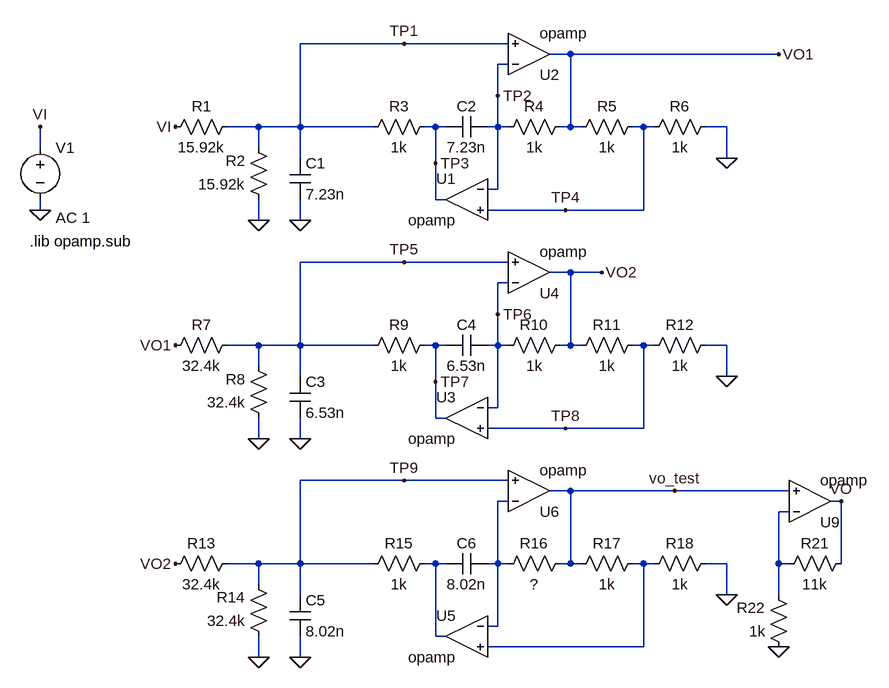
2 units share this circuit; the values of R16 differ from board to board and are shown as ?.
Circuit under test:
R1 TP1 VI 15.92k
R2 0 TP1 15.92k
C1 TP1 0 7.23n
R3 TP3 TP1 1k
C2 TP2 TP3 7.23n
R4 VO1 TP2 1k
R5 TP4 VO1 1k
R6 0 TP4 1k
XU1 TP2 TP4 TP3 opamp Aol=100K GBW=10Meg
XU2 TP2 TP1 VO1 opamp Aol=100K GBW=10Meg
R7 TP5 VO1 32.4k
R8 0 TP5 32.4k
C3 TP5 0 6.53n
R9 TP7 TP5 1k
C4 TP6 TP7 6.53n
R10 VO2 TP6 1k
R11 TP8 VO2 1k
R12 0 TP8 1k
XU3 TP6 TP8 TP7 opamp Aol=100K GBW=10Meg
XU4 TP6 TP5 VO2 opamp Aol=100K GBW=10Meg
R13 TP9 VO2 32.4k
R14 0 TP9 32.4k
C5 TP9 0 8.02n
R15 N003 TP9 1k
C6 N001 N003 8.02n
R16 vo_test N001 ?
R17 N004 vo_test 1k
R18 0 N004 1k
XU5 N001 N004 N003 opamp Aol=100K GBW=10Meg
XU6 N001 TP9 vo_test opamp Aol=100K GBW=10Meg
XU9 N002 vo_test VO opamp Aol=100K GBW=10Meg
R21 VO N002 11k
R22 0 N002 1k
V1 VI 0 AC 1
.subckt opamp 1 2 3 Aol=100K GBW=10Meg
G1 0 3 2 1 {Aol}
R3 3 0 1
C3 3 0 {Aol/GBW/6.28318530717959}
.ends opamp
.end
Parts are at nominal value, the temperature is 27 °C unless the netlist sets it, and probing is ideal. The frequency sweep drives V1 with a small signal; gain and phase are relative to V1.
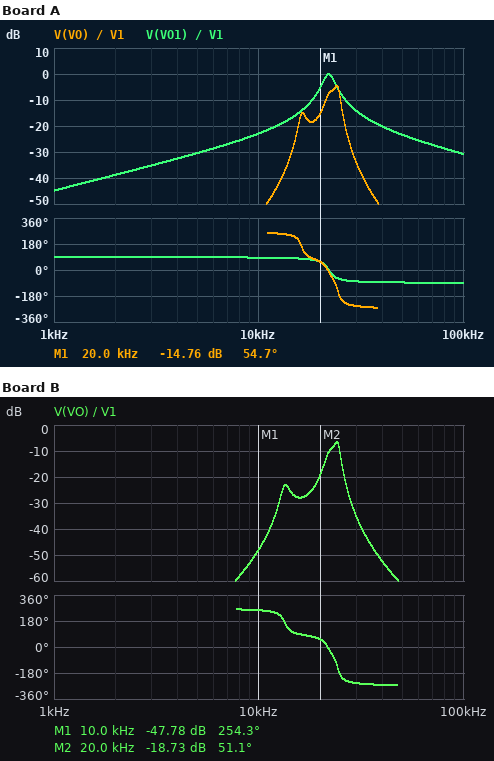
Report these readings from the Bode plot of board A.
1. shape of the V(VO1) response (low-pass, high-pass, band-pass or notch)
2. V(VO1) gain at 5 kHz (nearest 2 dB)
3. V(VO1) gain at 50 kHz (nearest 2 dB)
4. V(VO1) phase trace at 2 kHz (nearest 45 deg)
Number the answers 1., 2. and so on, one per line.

1. band-pass
2. -30 dB
3. -24 dB
4. 90 deg
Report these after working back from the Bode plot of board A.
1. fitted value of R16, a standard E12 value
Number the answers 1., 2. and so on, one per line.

1. 1.5 kΩ
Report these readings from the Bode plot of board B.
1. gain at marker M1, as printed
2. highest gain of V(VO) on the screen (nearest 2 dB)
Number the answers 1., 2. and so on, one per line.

1. -47.78 dB
2. -6 dB
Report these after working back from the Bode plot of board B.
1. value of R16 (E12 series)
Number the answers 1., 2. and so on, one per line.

1. 2.2 kΩ
